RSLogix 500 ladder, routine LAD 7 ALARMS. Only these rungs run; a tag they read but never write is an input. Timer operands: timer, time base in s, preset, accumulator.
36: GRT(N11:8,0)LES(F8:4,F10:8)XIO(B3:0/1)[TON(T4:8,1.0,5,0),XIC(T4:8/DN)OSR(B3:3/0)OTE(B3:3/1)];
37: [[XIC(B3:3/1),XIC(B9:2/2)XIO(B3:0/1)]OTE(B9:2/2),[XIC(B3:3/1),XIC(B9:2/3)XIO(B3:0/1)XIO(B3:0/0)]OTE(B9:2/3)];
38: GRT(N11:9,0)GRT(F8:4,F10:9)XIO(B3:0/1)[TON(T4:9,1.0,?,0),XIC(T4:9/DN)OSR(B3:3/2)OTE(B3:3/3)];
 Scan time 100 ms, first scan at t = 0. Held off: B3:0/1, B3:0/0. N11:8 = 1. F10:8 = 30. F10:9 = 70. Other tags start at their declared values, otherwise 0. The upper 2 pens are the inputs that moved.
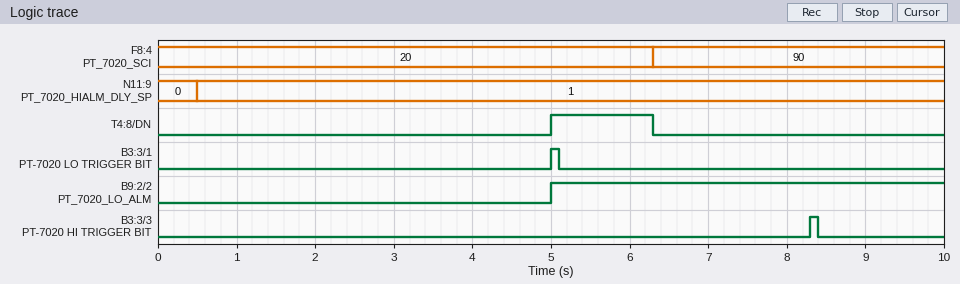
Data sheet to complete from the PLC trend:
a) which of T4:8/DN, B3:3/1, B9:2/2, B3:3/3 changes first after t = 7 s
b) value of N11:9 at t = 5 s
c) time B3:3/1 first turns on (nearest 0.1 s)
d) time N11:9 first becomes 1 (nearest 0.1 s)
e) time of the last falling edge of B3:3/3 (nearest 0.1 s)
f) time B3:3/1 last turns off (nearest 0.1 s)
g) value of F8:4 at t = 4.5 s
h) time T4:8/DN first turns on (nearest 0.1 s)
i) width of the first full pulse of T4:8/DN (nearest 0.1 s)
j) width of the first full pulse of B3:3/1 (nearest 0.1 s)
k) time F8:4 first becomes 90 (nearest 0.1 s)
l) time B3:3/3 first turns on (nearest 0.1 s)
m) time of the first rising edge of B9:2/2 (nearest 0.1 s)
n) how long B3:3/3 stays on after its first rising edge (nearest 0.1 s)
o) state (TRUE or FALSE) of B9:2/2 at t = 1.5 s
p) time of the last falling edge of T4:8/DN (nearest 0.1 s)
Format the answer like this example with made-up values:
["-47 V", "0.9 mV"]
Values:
["B3:3/3", "1", "5.0 s", "0.5 s", "8.4 s", "5.1 s", "20", "5.0 s", "1.3 s", "0.1 s", "6.3 s", "8.3 s", "5.0 s", "0.1 s", "FALSE", "6.3 s"]
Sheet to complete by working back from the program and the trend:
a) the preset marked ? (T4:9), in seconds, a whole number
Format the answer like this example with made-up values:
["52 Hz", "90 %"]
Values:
["2 s"]
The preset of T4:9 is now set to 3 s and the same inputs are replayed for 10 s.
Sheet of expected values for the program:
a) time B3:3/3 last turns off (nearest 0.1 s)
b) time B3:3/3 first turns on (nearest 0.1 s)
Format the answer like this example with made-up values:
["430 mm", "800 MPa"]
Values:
["9.4 s", "9.3 s"]
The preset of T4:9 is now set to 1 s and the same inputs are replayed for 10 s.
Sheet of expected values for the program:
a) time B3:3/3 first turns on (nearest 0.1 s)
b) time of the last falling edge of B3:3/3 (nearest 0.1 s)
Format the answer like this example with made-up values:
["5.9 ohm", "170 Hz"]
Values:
["7.3 s", "7.4 s"]
